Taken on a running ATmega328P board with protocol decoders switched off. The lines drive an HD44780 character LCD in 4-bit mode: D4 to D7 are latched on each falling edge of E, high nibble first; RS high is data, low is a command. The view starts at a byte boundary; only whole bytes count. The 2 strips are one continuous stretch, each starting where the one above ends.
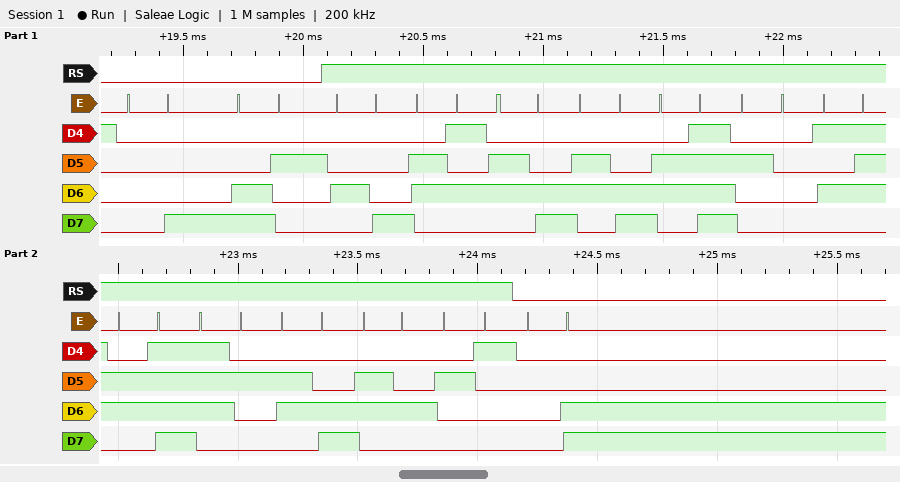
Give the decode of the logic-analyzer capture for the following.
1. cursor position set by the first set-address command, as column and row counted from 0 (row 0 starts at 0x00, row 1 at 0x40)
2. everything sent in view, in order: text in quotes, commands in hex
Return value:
column 2, row 1
0x08 0xC2 "Hello World!" 0x0C
